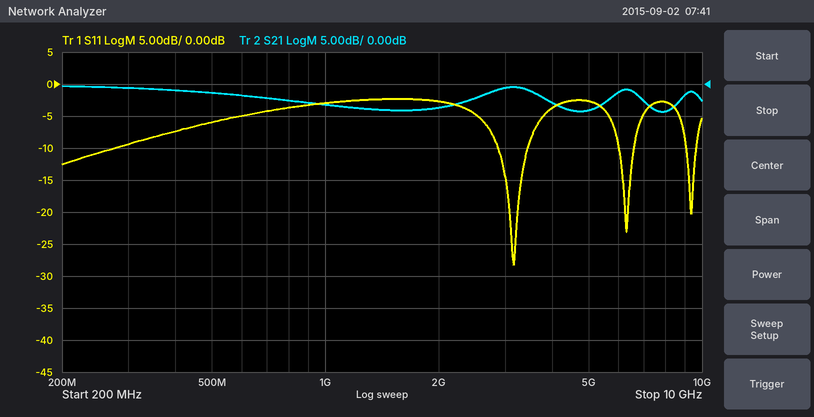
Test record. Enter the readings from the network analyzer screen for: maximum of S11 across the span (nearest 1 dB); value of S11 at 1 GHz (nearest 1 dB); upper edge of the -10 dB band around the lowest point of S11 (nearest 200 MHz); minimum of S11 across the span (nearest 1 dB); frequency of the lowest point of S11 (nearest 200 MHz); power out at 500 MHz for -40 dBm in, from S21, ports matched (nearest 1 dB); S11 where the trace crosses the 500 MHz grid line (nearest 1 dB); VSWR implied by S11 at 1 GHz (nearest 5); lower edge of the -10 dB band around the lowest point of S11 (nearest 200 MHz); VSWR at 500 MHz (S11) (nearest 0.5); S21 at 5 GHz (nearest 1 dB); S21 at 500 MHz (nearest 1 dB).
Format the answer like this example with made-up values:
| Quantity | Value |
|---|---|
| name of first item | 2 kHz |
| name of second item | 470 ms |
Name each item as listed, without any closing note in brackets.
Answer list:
| Quantity | Value |
|---|---|
| maximum of S11 across the span | -2 dB |
| value of S11 at 1 GHz | -3 dB |
| upper edge of the -10 dB band around the lowest point of S11 | 3.4 GHz |
| minimum of S11 across the span | -28 dB |
| frequency of the lowest point of S11 | 3.2 GHz |
| power out at 500 MHz for -40 dBm in, from S21, ports matched | -41 dBm |
| S11 where the trace crosses the 500 MHz grid line | -6 dB |
| VSWR implied by S11 at 1 GHz | 5 |
| lower edge of the -10 dB band around the lowest point of S11 | 2.8 GHz |
| VSWR at 500 MHz (S11) | 3.0 |
| S21 at 5 GHz | -4 dB |
| S21 at 500 MHz | -1 dB |
